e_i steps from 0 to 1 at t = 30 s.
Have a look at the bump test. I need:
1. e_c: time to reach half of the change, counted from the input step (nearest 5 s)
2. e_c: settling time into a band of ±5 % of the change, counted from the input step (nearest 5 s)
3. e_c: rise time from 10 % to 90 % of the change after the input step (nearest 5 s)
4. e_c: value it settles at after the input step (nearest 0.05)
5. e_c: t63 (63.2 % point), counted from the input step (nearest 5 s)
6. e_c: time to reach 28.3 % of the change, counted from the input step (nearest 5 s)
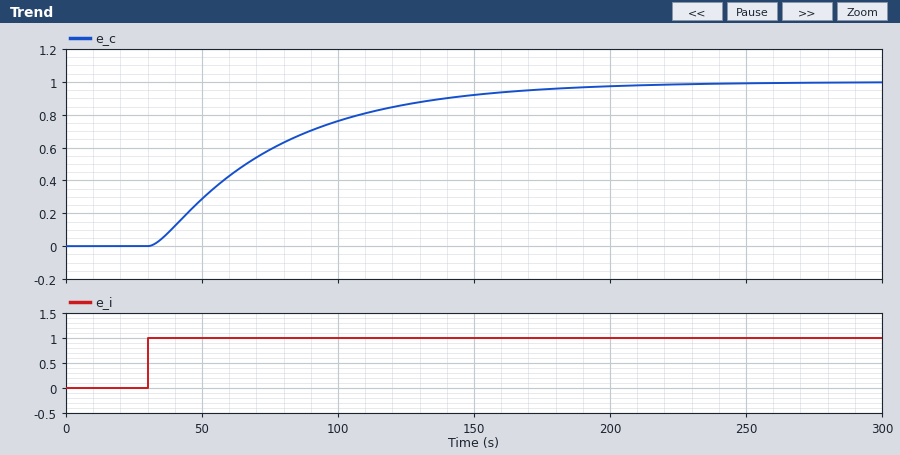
35 s
140 s
100 s
1.00
50 s
20 s
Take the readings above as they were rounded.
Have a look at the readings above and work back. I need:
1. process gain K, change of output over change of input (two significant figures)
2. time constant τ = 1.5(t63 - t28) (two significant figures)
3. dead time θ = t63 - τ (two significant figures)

1.0
45 s
5.0 s
